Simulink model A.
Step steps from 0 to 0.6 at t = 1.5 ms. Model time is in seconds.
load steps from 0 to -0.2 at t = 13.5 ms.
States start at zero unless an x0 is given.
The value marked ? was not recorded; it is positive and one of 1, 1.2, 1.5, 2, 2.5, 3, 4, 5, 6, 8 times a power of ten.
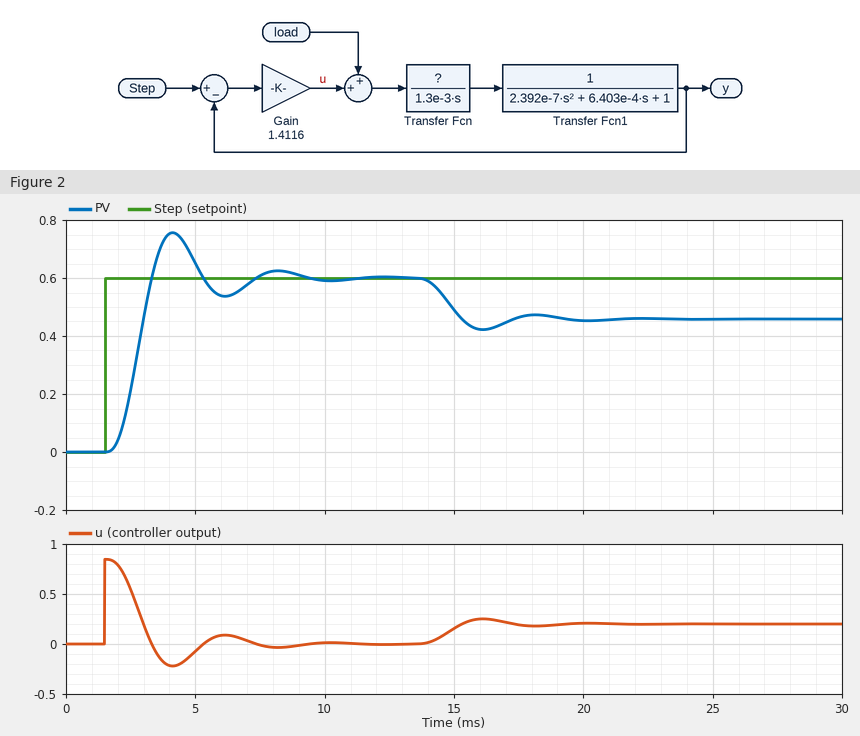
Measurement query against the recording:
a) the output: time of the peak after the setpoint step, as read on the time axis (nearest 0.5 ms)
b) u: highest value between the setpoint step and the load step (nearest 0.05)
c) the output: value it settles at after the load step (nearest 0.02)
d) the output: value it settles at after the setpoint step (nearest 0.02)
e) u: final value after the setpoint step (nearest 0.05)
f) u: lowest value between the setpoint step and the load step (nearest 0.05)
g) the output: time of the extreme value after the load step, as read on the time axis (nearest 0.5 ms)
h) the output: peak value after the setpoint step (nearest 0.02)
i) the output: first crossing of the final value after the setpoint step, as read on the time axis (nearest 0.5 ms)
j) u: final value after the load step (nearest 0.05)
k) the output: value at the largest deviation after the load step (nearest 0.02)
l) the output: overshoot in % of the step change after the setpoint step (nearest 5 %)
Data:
4.0 ms
0.85
0.46
0.60
0.00
-0.20
16.0 ms
0.76
3.5 ms
0.20
0.42
25 %
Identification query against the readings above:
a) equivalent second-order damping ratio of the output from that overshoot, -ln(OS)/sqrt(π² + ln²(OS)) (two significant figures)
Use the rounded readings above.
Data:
0.40
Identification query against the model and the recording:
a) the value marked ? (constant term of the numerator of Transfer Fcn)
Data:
1
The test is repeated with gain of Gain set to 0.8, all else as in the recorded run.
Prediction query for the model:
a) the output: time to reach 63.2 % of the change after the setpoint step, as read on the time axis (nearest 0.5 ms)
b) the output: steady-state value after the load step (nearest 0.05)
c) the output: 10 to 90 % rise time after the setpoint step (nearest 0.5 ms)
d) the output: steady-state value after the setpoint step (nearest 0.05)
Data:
3.5 ms
0.35
2.0 ms
0.60
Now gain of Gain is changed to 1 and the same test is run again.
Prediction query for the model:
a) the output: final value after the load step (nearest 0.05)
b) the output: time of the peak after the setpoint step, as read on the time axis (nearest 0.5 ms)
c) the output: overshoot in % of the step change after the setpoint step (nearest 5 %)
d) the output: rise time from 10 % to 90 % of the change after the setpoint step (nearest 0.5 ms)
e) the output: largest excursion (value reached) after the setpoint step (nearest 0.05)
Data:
0.40
4.5 ms
10 %
1.5 ms
0.65
